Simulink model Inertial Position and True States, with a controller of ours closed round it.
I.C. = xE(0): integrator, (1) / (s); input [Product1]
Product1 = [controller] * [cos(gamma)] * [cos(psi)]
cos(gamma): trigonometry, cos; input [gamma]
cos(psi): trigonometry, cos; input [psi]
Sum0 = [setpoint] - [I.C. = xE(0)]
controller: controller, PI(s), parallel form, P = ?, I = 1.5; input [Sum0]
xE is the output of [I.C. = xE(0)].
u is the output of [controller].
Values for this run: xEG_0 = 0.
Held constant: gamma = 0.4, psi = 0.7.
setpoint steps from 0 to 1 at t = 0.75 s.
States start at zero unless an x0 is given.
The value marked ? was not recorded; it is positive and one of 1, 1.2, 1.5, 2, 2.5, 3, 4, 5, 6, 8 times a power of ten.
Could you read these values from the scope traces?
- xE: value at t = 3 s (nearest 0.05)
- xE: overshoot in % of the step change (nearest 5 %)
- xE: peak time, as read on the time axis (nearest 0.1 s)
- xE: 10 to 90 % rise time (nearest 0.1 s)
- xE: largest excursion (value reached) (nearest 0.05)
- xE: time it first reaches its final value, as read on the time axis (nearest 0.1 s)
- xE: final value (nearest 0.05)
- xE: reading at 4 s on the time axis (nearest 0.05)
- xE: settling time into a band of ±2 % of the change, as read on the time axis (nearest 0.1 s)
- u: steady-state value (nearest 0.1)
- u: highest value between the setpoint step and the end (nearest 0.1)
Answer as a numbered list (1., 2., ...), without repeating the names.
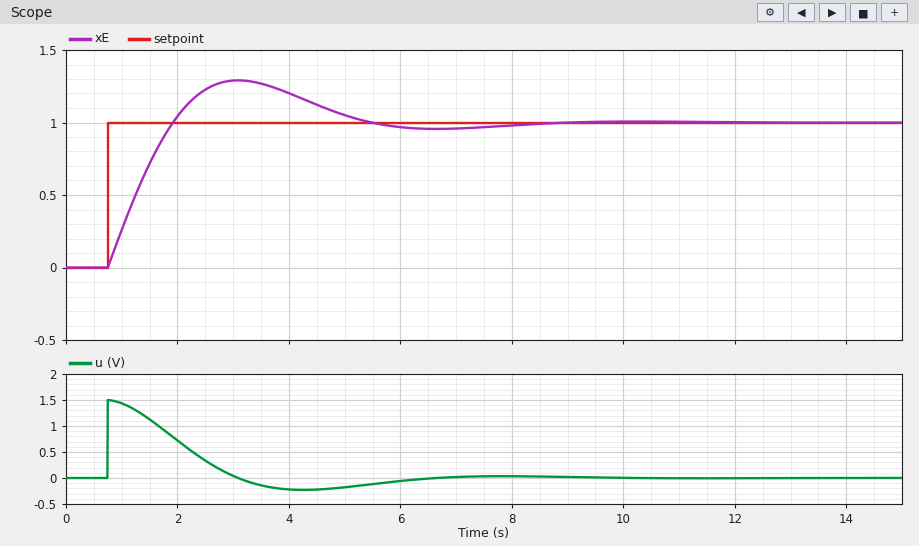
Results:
1. 1.30
2. 30 %
3. 3.1 s
4. 0.9 s
5. 1.30
6. 1.9 s
7. 1.00
8. 1.20
9. 8.0 s
10. 0.0
11. 1.5
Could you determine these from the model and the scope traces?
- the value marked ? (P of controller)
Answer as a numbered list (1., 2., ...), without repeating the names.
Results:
1. 1.5
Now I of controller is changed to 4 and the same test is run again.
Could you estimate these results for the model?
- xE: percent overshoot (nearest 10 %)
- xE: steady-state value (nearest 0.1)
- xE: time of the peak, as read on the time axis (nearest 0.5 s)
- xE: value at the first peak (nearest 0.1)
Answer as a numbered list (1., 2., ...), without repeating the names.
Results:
1. 40 %
2. 1.0
3. 2.5 s
4. 1.4
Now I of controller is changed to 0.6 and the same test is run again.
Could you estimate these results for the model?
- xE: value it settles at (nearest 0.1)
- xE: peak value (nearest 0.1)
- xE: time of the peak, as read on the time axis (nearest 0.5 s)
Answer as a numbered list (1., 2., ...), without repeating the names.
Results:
1. 1.0
2. 1.2
3. 4.0 s
